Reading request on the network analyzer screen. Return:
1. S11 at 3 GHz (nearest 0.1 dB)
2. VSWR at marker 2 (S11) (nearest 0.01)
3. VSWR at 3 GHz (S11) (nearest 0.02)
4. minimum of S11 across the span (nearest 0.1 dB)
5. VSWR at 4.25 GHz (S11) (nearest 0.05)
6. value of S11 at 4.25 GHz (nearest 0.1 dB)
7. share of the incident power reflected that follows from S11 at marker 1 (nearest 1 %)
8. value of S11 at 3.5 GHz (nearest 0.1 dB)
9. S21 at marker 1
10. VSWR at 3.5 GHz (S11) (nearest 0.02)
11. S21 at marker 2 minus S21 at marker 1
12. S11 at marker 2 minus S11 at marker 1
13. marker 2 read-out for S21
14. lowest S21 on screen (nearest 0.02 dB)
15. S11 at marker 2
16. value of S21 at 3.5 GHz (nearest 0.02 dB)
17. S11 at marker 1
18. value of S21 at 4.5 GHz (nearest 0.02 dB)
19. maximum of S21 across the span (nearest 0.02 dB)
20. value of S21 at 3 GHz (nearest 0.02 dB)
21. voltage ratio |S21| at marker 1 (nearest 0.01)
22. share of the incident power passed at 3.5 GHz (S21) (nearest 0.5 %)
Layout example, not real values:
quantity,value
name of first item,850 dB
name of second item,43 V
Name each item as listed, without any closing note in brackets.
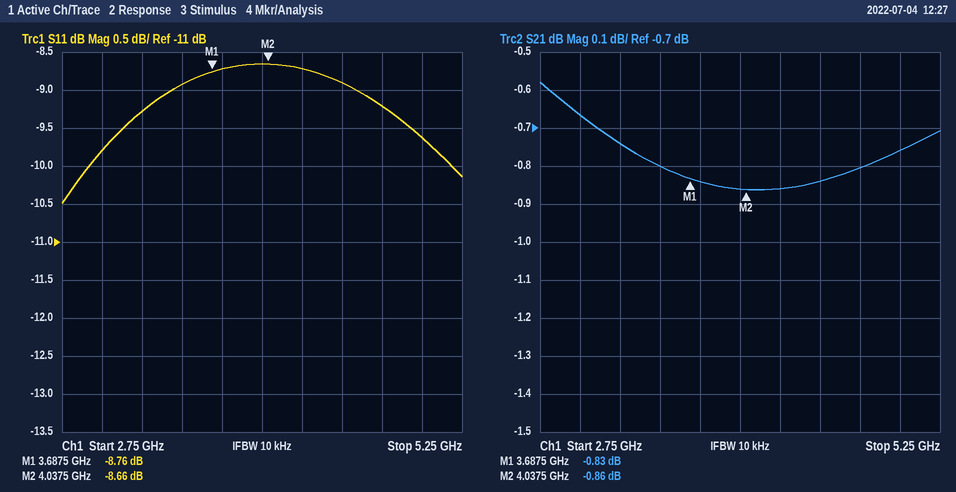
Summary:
quantity,value
S11 at 3 GHz,-9.8 dB
VSWR at marker 2 (S11),2.17
VSWR at 3 GHz (S11),1.96
minimum of S11 across the span,-10.5 dB
VSWR at 4.25 GHz (S11),2.15
value of S11 at 4.25 GHz,-8.7 dB
share of the incident power reflected that follows from S11 at marker 1,13 %
value of S11 at 3.5 GHz,-8.9 dB
S21 at marker 1,-0.83 dB
VSWR at 3.5 GHz (S11),2.12
S21 at marker 2 minus S21 at marker 1,-0.03 dB
S11 at marker 2 minus S11 at marker 1,0.10 dB
marker 2 read-out for S21,-0.86 dB
lowest S21 on screen,-0.86 dB
S11 at marker 2,-8.66 dB
value of S21 at 3.5 GHz,-0.80 dB
S11 at marker 1,-8.76 dB
value of S21 at 4.5 GHz,-0.84 dB
maximum of S21 across the span,-0.58 dB
value of S21 at 3 GHz,-0.66 dB
voltage ratio |S21| at marker 1,0.91
share of the incident power passed at 3.5 GHz (S21),83.0 %
